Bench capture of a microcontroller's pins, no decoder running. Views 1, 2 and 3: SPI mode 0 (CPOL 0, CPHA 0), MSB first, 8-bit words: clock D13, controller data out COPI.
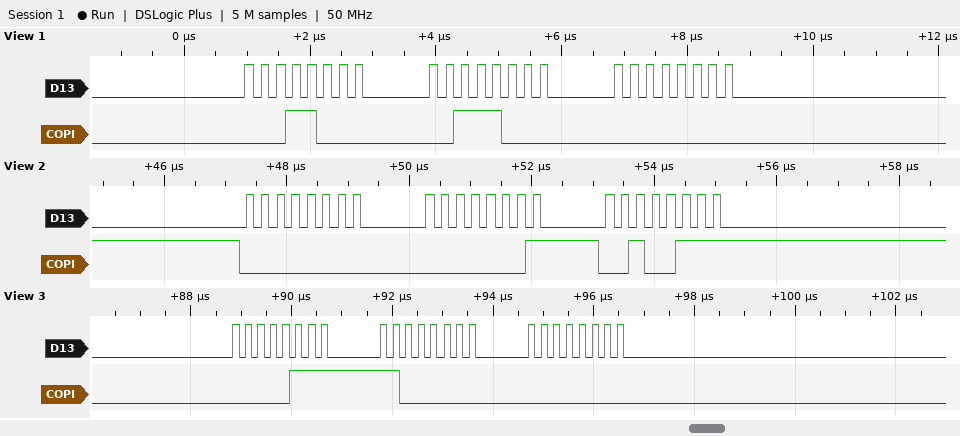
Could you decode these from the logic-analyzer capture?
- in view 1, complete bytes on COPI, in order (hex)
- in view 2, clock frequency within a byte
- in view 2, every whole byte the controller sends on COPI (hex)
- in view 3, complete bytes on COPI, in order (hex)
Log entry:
18 38 00
4 MHz
00 01 27
07 C0 00
